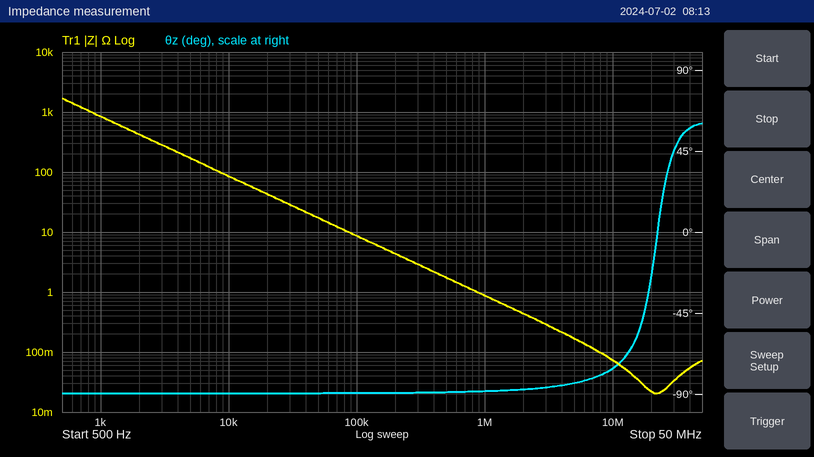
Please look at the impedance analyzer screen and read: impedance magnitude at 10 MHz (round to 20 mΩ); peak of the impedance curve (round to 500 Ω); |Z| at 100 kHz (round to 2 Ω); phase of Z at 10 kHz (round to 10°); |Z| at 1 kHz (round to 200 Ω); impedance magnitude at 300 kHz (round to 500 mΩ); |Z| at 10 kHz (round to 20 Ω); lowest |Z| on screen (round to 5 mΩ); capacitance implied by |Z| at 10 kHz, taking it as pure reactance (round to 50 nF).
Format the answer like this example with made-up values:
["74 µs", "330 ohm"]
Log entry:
["80 mΩ", "1.5 kΩ", "8 Ω", "-90°", "800 Ω", "3.0 Ω", "80 Ω", "20 mΩ", "200 nF"]
